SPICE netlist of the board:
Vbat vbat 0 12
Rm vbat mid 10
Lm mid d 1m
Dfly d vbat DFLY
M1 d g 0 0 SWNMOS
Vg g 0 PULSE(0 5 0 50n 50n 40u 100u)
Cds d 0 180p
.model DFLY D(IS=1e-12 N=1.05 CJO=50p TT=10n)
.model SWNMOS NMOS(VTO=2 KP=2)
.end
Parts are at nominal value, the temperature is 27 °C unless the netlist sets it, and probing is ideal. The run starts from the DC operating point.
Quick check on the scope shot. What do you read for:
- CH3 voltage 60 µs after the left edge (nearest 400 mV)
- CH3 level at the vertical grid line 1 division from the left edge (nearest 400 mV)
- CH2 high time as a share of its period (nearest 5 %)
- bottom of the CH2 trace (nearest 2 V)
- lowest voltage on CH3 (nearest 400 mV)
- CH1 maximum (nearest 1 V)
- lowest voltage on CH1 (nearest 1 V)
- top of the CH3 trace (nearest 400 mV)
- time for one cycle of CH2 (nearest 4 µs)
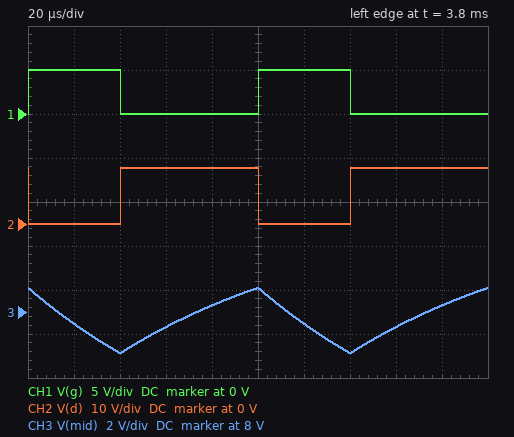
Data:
7.2 V
7.6 V
60 %
0 V
6.0 V
5 V
0 V
9.2 V
100 µs
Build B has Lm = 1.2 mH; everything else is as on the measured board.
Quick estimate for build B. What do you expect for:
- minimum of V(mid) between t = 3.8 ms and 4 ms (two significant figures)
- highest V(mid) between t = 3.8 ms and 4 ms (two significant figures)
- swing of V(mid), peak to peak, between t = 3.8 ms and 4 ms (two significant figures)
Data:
6.4 V
8.9 V
2.5 V
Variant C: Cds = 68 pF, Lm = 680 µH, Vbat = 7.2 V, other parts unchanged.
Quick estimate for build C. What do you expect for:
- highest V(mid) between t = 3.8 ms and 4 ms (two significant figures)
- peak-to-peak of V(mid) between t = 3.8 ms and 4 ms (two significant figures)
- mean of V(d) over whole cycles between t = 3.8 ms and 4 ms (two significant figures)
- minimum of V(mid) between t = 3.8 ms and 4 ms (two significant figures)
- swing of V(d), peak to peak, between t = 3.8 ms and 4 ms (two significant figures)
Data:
6.0 V
2.7 V
4.8 V
3.4 V
7.9 V
